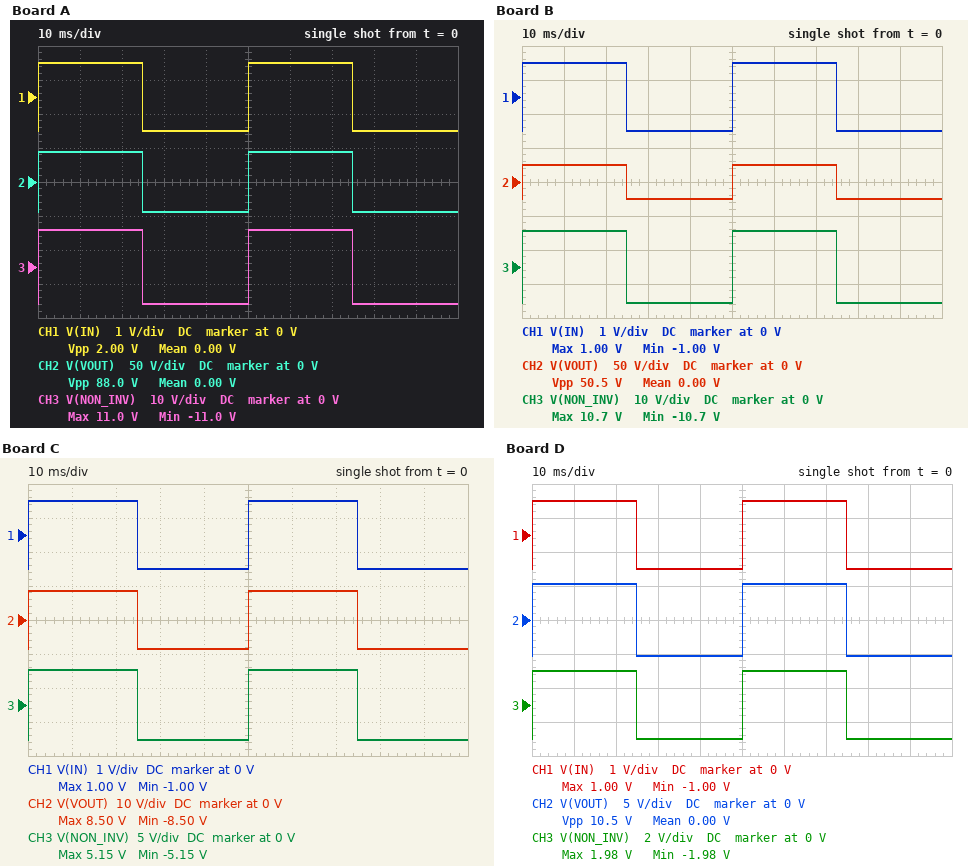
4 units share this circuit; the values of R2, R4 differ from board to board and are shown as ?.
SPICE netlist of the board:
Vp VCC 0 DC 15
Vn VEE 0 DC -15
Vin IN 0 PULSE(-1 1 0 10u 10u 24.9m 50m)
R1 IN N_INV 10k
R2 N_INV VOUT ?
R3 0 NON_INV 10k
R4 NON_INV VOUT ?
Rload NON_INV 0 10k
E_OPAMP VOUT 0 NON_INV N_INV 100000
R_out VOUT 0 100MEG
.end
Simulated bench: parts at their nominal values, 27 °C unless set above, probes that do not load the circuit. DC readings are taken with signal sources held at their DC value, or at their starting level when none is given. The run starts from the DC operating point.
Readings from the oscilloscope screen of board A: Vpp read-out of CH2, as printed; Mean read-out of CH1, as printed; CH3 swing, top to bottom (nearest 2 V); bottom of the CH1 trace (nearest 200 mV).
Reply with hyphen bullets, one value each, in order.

- 88.0 V
- 0.00 V
- 22 V
- -1.0 V
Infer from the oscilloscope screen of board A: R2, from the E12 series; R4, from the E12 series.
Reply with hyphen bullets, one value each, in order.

- 33 kΩ
- 15 kΩ
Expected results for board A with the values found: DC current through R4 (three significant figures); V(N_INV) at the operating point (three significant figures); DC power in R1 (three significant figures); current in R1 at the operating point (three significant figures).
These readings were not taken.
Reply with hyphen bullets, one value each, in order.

- 2.20 mA
- -11.0 V
- 10.0 mW
- 1.00 mA
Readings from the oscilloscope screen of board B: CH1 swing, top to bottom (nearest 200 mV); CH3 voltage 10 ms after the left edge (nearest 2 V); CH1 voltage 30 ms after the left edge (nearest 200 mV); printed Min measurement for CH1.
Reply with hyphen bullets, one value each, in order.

- 2.0 V
- 10 V
- -1.0 V
- -1.00 V
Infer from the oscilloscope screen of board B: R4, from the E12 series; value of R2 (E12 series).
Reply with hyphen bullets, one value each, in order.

- 6.8 kΩ
- 15 kΩ
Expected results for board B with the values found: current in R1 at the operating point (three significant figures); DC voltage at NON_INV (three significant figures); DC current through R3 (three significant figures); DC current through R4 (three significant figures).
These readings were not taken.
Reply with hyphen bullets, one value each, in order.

- 972 µA
- -10.7 V
- 1.07 mA
- 2.14 mA
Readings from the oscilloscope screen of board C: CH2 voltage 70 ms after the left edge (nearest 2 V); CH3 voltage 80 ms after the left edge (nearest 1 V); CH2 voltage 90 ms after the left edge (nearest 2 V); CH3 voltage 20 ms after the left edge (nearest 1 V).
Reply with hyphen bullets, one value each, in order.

- 8 V
- -5 V
- -8 V
- 5 V
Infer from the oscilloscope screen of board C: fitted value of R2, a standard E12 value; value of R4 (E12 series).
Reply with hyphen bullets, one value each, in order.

- 8.2 kΩ
- 3.3 kΩ
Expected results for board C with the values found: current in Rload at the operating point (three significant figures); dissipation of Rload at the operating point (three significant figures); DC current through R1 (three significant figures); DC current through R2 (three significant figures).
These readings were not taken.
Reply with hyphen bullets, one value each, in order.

- 513 µA
- 2.63 mW
- 413 µA
- 413 µA
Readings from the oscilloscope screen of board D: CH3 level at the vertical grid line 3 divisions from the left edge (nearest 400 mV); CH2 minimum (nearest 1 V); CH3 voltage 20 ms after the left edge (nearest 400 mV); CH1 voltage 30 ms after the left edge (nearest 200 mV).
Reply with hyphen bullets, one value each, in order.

- -2.0 V
- -5 V
- 2.0 V
- -1.0 V
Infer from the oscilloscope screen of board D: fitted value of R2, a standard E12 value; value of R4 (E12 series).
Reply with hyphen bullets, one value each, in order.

- 33 kΩ
- 8.2 kΩ
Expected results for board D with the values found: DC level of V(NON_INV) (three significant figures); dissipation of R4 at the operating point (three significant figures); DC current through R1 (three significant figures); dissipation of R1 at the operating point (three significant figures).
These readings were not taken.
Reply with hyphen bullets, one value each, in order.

- -1.99 V
- 1.30 mW
- 98.8 µA
- 97.6 µW
